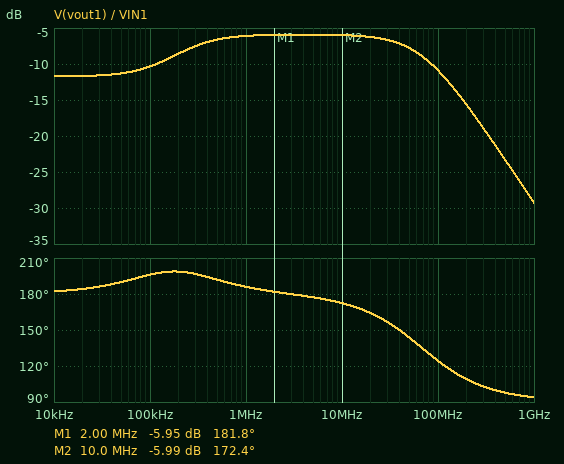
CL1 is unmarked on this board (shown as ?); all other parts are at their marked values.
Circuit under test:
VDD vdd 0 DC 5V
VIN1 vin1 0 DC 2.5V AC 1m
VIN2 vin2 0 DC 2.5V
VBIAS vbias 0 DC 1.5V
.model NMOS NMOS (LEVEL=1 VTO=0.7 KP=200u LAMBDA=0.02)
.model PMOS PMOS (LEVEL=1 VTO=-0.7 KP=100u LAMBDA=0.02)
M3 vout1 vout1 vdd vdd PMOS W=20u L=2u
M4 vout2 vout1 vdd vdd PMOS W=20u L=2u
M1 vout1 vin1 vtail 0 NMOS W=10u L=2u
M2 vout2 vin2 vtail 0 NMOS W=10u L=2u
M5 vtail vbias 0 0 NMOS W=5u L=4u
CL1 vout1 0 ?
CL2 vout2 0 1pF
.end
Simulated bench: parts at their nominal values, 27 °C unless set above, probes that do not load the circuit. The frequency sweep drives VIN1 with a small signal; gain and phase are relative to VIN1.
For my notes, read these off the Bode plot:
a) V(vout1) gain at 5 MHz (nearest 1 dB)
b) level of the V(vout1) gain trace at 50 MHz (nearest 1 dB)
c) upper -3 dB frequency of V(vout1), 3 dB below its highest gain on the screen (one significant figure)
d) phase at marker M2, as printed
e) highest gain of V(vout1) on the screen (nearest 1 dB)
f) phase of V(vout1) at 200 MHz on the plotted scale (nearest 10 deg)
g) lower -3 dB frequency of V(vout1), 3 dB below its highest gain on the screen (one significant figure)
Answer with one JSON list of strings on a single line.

["-6 dB", "-8 dB", "70 MHz", "172.4 deg", "-6 dB", "110 deg", "200 kHz"]
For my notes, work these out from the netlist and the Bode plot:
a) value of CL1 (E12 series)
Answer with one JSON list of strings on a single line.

["680 fF"]
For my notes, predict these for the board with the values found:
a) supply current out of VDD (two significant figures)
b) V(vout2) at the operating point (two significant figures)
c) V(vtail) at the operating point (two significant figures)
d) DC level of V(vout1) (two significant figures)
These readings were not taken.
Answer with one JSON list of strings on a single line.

["82 µA", "4.0 V", "1.5 V", "4.0 V"]
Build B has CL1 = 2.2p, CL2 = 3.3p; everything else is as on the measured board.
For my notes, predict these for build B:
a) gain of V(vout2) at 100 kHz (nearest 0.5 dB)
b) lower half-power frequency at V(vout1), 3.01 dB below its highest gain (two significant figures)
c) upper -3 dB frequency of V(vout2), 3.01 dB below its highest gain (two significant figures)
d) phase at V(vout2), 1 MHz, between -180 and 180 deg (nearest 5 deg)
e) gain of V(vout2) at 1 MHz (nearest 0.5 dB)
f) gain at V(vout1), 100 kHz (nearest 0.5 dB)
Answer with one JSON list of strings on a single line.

["41.0 dB", "53 kHz", "77 kHz", "-85 deg", "23.0 dB", "-7.5 dB"]
